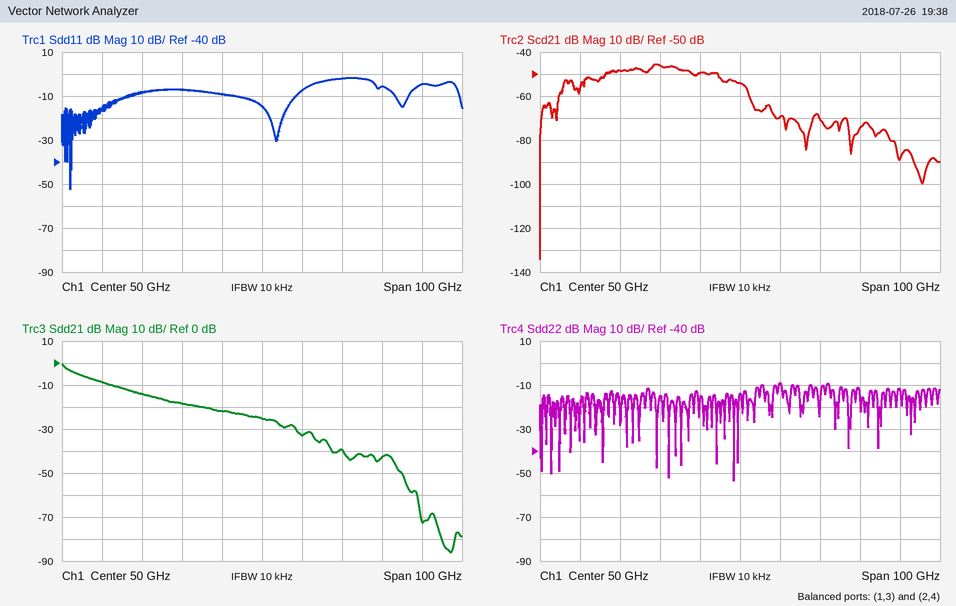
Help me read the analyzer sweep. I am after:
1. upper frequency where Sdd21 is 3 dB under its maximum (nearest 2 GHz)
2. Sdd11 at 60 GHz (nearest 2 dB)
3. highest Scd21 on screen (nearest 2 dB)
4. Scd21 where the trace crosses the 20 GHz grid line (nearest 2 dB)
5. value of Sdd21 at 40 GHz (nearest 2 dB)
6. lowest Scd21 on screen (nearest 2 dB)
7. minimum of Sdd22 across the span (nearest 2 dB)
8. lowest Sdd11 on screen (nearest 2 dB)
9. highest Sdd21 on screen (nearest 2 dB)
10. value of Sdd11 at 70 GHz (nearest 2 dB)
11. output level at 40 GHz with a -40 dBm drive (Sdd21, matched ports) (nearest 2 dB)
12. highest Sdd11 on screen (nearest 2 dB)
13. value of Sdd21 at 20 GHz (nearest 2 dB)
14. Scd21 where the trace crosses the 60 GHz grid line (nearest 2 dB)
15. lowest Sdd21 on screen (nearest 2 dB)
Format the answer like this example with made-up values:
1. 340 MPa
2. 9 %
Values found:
1. 2 GHz
2. -8 dB
3. -46 dB
4. -48 dB
5. -22 dB
6. -134 dB
7. -54 dB
8. -52 dB
9. 0 dB
10. -2 dB
11. -62 dBm
12. -2 dB
13. -14 dB
14. -70 dB
15. -86 dB
